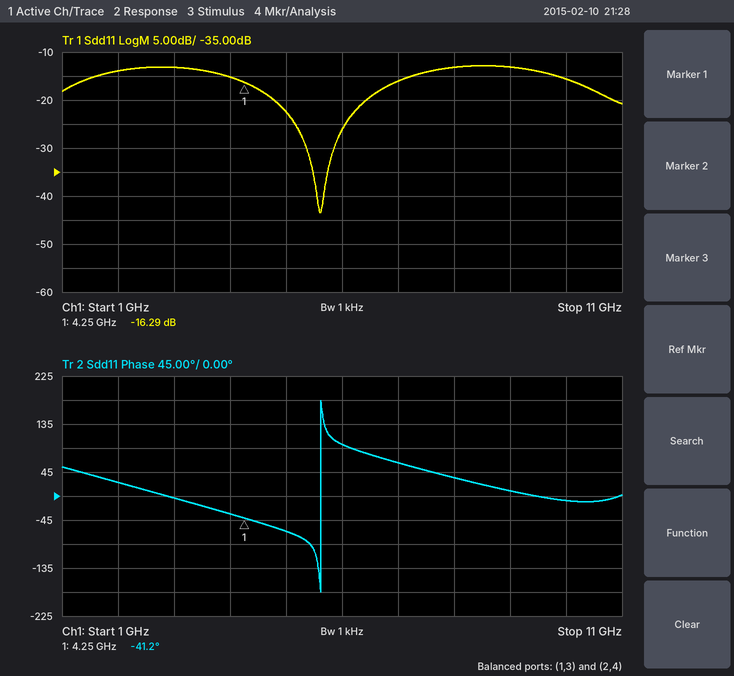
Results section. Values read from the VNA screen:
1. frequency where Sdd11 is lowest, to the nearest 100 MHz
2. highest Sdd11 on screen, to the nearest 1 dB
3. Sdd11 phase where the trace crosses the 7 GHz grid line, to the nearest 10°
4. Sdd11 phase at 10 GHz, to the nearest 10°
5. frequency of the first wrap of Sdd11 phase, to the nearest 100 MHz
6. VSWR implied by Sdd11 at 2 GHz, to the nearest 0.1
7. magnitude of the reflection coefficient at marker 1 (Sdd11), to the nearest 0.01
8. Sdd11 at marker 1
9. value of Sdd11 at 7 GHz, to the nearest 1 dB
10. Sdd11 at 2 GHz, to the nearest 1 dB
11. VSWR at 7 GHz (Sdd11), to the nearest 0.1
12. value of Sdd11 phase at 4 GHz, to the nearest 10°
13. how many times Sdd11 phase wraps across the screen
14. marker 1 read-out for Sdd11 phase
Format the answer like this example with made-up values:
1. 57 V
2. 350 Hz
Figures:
1. 5.6 GHz
2. -13 dB
3. 60°
4. -10°
5. 5.6 GHz
6. 1.5
7. 0.15
8. -16.29 dB
9. -16 dB
10. -14 dB
11. 1.4
12. -30°
13. 1
14. -41.2°
